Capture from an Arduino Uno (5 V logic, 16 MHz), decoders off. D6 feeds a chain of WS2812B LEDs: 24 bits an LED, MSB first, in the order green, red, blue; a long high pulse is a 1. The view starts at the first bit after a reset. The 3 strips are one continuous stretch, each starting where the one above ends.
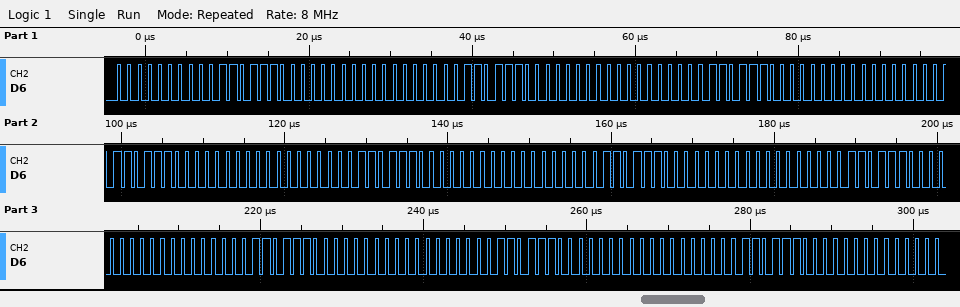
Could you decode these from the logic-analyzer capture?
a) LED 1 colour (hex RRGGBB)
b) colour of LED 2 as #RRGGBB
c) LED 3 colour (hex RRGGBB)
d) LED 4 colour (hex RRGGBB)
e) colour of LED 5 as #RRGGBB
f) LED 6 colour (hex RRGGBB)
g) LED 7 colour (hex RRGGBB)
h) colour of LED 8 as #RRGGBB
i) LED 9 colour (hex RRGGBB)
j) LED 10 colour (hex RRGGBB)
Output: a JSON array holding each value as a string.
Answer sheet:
["#370000", "#370000", "#370000", "#370000", "#370000", "#370000", "#370000", "#370000", "#370000", "#370000"]
